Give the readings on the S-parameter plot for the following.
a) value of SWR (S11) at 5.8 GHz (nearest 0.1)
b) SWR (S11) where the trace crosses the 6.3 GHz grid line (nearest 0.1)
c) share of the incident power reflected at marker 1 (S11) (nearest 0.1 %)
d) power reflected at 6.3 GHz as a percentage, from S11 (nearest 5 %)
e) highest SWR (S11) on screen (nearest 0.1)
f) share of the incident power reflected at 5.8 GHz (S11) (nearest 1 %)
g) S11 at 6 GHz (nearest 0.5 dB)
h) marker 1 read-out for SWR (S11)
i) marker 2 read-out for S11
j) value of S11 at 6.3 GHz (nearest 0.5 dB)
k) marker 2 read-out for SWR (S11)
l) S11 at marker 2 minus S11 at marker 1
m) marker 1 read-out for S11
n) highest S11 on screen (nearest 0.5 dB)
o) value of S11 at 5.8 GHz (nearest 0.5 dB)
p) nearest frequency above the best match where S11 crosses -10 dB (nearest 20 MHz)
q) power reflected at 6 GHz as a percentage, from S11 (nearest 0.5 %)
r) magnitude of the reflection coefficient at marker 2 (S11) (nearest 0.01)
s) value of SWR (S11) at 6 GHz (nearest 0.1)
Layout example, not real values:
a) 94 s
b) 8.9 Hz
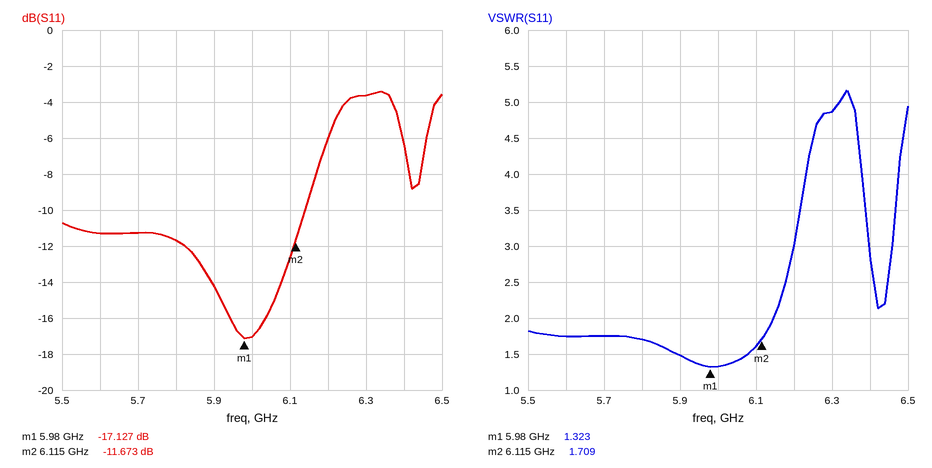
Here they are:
a) 1.7
b) 4.9
c) 1.9 %
d) 45 %
e) 5.2
f) 7 %
g) -17.0 dB
h) 1.323
i) -11.673 dB
j) -3.5 dB
k) 1.709
l) 5.454 dB
m) -17.127 dB
n) -3.5 dB
o) -11.5 dB
p) 6.14 GHz
q) 2.0 %
r) 0.26
s) 1.3
